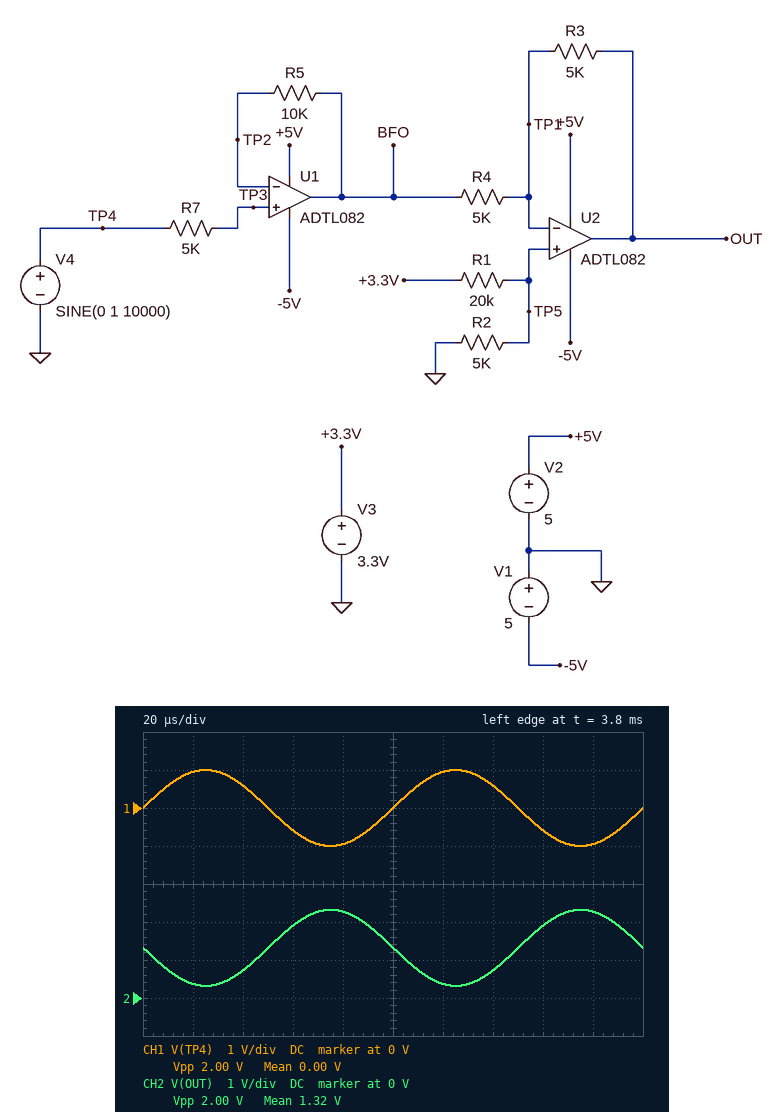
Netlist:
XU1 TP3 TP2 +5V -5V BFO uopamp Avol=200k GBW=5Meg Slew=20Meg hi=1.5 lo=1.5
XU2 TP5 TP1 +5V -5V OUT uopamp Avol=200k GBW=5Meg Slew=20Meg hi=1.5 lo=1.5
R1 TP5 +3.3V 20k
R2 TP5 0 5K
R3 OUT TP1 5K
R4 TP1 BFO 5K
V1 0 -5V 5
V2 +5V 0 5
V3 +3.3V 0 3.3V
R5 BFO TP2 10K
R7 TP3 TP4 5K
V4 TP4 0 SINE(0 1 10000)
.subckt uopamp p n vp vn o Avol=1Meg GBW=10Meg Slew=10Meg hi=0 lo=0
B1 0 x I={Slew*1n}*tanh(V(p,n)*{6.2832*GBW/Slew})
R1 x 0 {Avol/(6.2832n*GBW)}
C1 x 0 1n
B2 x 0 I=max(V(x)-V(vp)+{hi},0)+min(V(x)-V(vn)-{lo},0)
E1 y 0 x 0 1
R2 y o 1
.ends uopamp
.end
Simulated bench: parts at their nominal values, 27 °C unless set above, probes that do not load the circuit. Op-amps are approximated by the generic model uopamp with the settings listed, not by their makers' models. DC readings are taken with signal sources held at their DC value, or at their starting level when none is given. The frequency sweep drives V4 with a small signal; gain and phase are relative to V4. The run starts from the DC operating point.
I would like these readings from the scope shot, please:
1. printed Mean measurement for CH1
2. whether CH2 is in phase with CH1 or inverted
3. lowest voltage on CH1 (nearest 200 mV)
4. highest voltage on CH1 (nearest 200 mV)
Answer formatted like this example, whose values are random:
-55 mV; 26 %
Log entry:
0.00 V; inverted; -1.0 V; 1.0 V
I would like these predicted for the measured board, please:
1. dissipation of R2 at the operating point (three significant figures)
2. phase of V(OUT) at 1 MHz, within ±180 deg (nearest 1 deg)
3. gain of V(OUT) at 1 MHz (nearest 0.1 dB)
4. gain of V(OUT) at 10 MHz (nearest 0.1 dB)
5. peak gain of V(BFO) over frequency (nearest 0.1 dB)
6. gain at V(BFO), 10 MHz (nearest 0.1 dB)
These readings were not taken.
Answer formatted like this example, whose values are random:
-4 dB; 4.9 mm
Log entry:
87.1 µW; 147 deg; -0.8 dB; -19.3 dB; 0 dB; -7.0 dB
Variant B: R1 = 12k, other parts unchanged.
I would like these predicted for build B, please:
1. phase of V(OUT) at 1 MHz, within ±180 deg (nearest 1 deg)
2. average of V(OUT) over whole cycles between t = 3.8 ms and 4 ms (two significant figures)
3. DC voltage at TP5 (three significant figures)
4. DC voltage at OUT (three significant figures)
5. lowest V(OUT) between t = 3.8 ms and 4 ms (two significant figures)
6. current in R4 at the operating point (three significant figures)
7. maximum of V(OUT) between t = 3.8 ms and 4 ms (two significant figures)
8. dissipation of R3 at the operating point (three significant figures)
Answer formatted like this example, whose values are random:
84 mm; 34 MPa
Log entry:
147 deg; 1.9 V; 971 mV; 1.94 V; 940 mV; 194 µA; 2.9 V; 188 µW
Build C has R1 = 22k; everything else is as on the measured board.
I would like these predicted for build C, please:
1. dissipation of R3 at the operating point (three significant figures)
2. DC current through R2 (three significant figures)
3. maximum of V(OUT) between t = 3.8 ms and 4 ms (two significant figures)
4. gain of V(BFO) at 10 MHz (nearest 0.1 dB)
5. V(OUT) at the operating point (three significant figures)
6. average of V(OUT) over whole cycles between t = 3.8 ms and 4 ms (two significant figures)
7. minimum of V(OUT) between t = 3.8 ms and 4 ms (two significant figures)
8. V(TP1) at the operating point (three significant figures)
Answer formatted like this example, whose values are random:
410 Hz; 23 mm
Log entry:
74.7 µW; 122 µA; 2.2 V; -7.0 dB; 1.22 V; 1.2 V; 220 mV; 611 mV
